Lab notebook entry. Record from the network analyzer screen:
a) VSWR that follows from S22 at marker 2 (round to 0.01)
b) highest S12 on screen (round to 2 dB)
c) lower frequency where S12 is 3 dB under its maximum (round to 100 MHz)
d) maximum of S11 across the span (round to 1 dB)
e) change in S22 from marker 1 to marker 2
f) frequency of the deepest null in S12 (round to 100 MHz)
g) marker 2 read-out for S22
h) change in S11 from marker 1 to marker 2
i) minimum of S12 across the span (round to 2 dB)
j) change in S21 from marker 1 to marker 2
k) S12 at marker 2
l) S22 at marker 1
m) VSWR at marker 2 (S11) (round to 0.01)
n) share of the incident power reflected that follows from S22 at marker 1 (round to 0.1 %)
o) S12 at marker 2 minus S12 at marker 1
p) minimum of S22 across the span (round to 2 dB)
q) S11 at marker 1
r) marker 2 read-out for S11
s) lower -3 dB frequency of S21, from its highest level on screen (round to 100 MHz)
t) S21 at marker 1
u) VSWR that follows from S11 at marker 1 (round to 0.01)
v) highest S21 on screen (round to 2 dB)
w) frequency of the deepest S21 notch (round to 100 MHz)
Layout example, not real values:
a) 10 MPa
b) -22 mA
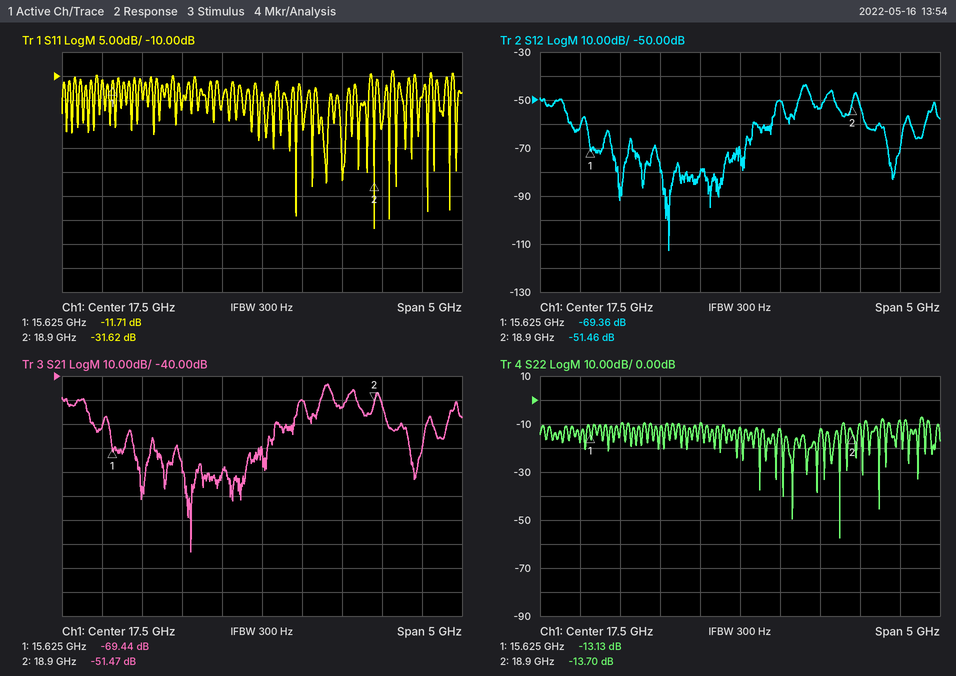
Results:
a) 1.52
b) -44 dB
c) 18.3 GHz
d) -9 dB
e) -0.57 dB
f) 16.6 GHz
g) -13.70 dB
h) -19.91 dB
i) -112 dB
j) 17.97 dB
k) -51.46 dB
l) -13.13 dB
m) 1.05
n) 4.9 %
o) 17.90 dB
p) -58 dB
q) -11.71 dB
r) -31.62 dB
s) 18.3 GHz
t) -69.44 dB
u) 1.70
v) -44 dB
w) 16.6 GHz
